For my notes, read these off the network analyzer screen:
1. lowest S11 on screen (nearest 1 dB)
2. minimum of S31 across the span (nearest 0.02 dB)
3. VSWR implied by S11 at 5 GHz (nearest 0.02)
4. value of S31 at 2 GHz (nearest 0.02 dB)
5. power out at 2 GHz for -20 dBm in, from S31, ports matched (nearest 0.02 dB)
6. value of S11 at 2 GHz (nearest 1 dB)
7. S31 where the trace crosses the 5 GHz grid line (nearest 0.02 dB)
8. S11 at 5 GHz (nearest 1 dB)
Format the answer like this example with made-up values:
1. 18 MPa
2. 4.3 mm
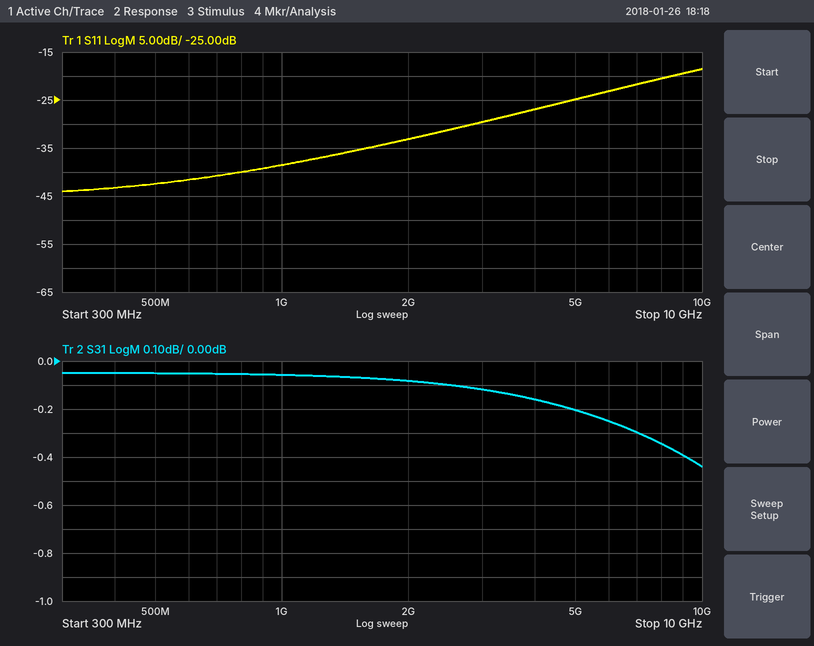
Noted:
1. -44 dB
2. -0.44 dB
3. 1.12
4. -0.08 dB
5. -20.08 dBm
6. -33 dB
7. -0.20 dB
8. -25 dB
